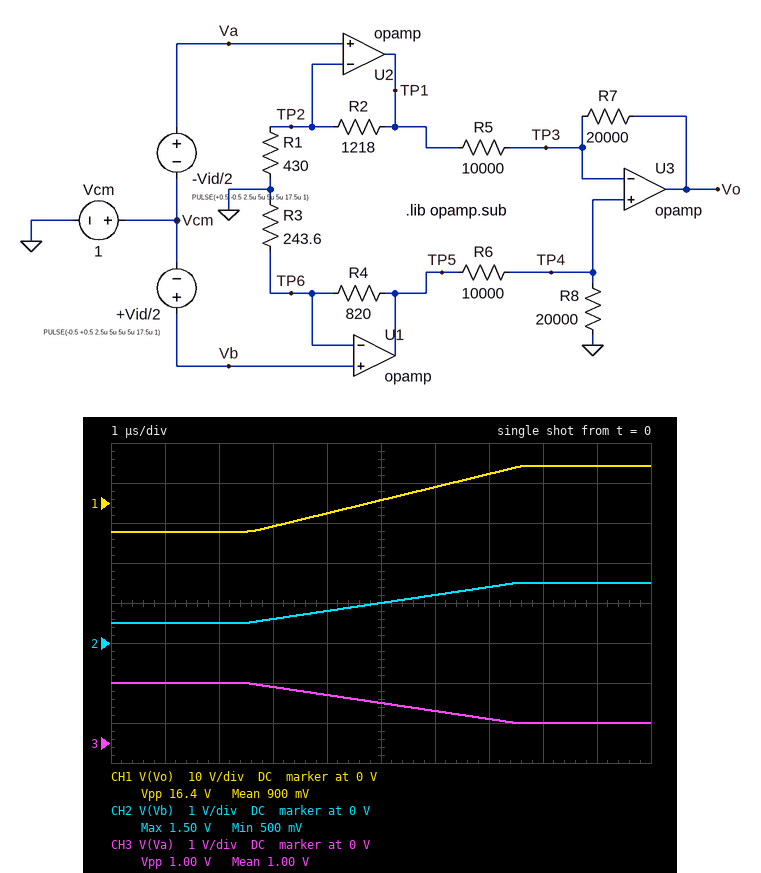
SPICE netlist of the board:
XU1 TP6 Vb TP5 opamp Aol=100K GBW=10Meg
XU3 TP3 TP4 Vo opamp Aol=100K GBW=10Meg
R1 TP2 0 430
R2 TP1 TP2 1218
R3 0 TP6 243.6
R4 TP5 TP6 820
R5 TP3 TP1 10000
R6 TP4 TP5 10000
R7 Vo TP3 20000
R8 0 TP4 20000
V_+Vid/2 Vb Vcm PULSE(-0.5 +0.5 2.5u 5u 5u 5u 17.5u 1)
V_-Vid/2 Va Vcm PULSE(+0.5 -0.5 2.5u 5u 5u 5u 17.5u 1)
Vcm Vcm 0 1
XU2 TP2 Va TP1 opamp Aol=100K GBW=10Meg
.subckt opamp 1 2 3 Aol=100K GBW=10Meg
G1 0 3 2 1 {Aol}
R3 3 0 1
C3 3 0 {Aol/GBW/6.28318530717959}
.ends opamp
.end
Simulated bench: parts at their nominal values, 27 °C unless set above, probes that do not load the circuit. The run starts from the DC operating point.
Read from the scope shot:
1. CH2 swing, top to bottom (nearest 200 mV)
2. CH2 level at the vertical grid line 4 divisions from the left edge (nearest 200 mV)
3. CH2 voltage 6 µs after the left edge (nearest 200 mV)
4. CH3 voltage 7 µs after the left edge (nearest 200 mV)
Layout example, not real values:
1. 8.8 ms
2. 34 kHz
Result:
1. 1.0 V
2. 800 mV
3. 1.2 V
4. 600 mV
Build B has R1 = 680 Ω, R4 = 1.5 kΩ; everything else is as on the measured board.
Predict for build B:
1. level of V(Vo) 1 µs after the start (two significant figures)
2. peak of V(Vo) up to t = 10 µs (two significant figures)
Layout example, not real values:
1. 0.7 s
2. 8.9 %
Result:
1. -1.2 V
2. 19 V
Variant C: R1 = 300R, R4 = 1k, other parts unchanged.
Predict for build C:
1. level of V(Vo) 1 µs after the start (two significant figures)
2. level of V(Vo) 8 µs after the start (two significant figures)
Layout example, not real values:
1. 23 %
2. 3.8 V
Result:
1. -10 V
2. 10 V
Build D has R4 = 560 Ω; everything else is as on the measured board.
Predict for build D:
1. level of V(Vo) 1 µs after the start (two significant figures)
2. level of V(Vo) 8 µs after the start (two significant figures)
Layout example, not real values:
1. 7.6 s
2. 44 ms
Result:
1. -8.2 V
2. 6.1 V
